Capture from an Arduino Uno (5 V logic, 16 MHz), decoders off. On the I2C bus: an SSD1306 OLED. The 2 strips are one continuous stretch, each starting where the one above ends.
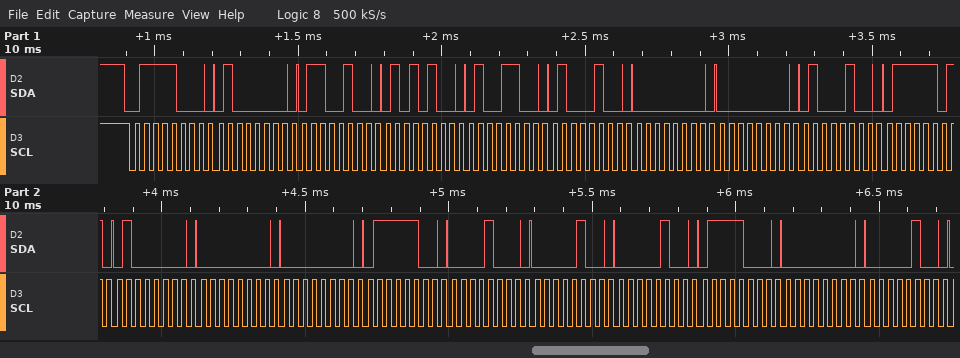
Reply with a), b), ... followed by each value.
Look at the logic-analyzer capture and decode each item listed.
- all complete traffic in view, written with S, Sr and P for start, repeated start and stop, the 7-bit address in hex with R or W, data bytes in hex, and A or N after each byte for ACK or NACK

a) S 3CW A 40 A 64 A 54 A 4C A 44 A 00 A 00 A 44 A 7D A 40 A 00 A 00 A 7C A 08 A 04 A 04 A 78 A 00 A 04 A
